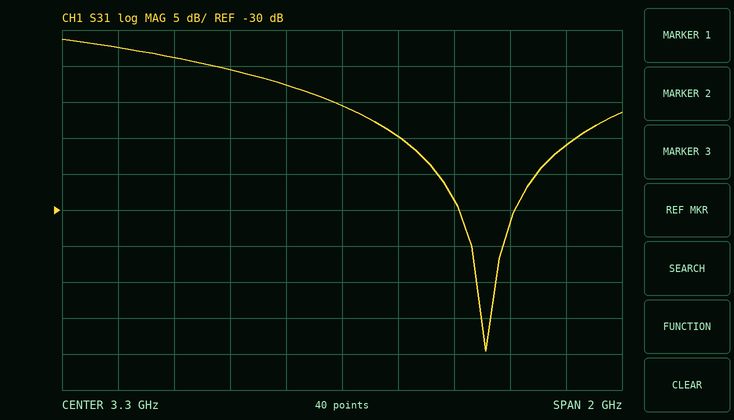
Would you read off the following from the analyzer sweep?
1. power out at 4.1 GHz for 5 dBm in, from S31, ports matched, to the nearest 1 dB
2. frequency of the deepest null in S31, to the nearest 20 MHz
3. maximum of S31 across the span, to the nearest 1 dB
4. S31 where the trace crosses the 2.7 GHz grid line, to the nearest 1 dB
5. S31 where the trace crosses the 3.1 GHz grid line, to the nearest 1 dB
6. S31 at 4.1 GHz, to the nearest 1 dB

-16 dBm
3.82 GHz
-6 dB
-9 dB
-13 dB
-21 dB
